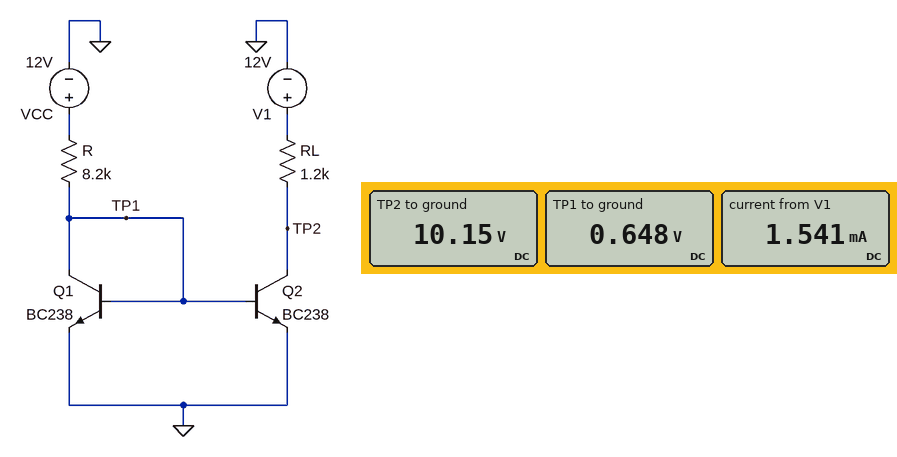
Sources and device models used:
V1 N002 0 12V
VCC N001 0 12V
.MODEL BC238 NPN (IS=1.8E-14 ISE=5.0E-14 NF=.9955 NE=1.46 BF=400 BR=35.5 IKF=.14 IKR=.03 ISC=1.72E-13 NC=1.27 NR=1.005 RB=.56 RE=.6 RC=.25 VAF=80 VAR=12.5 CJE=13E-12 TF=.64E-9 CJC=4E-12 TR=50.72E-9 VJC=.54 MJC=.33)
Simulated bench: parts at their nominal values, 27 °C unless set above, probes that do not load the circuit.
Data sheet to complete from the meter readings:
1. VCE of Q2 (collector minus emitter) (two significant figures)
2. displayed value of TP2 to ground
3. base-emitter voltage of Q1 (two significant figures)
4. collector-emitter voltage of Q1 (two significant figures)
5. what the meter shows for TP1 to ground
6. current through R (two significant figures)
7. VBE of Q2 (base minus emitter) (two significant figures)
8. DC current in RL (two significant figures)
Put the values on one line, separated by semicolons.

10 V; 10.15 V; 650 mV; 650 mV; 0.648 V; 1.4 mA; 650 mV; 1.5 mA
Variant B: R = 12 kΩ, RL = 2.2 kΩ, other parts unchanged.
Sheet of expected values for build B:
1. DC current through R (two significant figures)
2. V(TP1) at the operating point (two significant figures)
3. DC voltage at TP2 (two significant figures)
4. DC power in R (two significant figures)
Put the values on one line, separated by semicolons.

950 µA; 640 mV; 9.7 V; 11 mW
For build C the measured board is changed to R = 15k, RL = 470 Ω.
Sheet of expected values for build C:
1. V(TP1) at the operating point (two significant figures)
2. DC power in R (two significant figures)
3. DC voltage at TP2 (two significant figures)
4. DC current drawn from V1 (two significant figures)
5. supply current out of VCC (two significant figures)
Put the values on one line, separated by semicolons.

630 mV; 8.6 mW; 12 V; 860 µA; 760 µA
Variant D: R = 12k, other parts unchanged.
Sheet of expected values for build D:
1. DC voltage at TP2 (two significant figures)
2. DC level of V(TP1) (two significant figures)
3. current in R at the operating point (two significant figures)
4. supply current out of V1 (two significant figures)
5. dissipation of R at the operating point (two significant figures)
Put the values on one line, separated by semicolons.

11 V; 640 mV; 950 µA; 1.1 mA; 11 mW
